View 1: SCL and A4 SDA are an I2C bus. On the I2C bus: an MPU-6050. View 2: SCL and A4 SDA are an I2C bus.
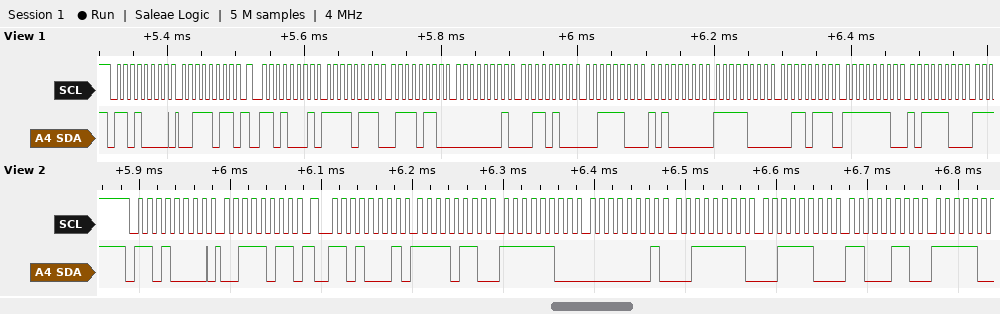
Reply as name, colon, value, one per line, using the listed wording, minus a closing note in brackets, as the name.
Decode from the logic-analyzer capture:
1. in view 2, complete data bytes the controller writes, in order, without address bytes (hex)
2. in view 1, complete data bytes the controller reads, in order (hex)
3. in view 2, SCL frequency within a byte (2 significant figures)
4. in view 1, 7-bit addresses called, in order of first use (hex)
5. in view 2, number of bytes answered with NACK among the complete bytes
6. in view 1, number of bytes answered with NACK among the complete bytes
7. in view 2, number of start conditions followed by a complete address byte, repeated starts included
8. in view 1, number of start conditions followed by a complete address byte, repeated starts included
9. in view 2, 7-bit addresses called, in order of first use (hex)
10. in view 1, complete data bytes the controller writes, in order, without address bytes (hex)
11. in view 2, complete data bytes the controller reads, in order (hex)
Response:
in view 2, complete data bytes the controller writes, in order, without address bytes: 3B
in view 1, complete data bytes the controller reads, in order: F7 76 01 34 3C A0 F8 37 FE BC
in view 2, SCL frequency within a byte: 100 kHz
in view 1, 7-bit addresses called, in order of first use: 0x68
in view 2, number of bytes answered with NACK among the complete bytes: 0
in view 1, number of bytes answered with NACK among the complete bytes: 0
in view 2, number of start conditions followed by a complete address byte, repeated starts included: 2
in view 1, number of start conditions followed by a complete address byte, repeated starts included: 2
in view 2, 7-bit addresses called, in order of first use: 0x68
in view 1, complete data bytes the controller writes, in order, without address bytes: 3B
in view 2, complete data bytes the controller reads, in order: F6 FC 01 3F 3C C6
